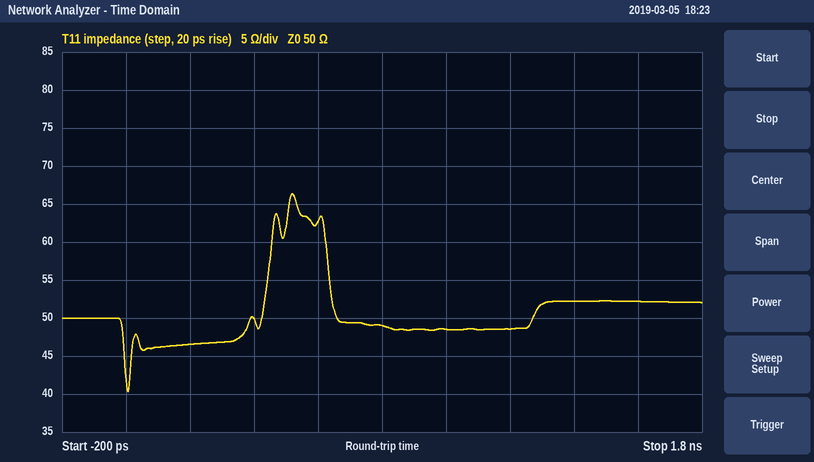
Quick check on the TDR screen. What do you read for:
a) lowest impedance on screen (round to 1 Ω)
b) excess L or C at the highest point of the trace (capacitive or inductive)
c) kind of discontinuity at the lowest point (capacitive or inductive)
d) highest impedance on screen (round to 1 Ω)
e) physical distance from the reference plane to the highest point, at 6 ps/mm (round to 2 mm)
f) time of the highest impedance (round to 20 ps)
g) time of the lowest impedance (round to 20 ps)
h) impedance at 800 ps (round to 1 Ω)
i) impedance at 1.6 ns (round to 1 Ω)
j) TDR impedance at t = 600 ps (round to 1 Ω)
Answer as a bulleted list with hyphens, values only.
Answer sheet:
- 40 Ω
- inductive
- capacitive
- 66 Ω
- 44 mm
- 520 ps
- 0 ps
- 49 Ω
- 52 Ω
- 63 Ω
